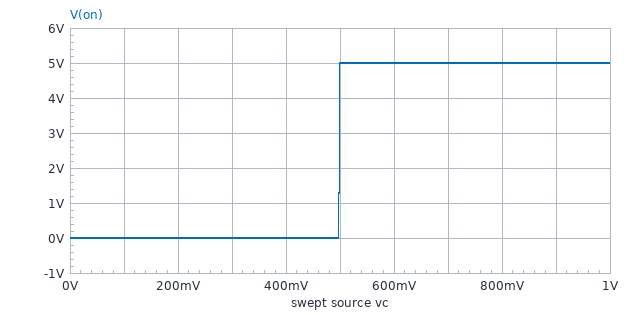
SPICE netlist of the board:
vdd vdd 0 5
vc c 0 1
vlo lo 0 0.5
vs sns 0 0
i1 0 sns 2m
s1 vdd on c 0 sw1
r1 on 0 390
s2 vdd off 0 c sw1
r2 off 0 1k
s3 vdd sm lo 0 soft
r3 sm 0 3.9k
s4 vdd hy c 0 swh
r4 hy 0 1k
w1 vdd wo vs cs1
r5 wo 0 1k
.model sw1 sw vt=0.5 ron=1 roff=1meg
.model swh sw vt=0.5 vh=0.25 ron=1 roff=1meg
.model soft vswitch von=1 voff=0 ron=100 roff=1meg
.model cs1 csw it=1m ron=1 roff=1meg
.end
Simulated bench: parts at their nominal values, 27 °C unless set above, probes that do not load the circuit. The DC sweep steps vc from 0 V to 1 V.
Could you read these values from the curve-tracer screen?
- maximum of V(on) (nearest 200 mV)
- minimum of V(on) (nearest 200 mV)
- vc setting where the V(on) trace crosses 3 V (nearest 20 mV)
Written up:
5.0 V
0 V
500 mV
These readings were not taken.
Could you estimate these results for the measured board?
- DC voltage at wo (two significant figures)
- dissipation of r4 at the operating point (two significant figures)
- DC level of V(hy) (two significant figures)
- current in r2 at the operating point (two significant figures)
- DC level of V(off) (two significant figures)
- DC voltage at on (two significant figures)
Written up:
5.0 V
25 mW
5.0 V
5.0 µA
5.0 mV
5.0 V
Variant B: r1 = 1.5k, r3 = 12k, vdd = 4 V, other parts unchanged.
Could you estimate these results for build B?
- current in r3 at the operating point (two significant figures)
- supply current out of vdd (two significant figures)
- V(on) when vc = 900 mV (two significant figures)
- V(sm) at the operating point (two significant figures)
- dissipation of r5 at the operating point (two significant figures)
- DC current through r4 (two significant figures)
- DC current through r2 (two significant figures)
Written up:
180 µA
11 mA
4.0 V
2.2 V
16 mW
4.0 mA
4.0 µA
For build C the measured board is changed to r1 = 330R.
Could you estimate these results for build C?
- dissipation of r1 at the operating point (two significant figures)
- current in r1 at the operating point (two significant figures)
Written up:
75 mW
15 mA
